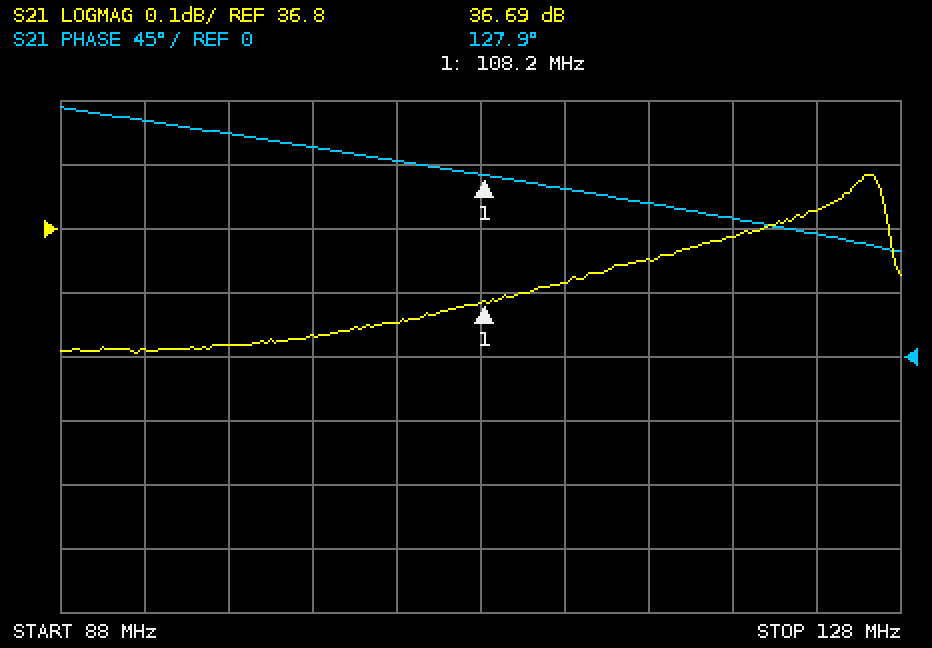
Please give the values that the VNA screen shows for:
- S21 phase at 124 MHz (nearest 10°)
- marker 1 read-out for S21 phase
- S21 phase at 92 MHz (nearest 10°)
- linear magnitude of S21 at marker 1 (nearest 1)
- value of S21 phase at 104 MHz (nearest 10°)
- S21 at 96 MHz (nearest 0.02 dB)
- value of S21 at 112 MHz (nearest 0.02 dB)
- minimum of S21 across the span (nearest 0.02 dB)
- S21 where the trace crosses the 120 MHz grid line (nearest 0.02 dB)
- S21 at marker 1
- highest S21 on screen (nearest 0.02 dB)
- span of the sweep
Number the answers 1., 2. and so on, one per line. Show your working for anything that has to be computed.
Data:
1. 90°
2. 127.9°
3. 170°
4. 10^(36.69/20) ≈ 68
5. 140°
6. 36.62 dB
7. 36.72 dB
8. 36.60 dB
9. 36.78 dB
10. 36.69 dB
11. 36.88 dB
12. 40 MHz
